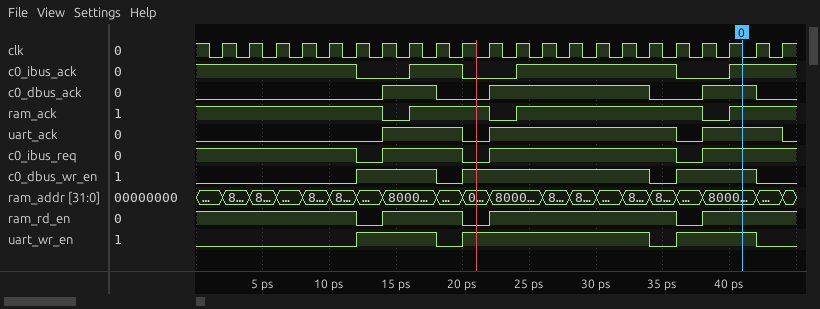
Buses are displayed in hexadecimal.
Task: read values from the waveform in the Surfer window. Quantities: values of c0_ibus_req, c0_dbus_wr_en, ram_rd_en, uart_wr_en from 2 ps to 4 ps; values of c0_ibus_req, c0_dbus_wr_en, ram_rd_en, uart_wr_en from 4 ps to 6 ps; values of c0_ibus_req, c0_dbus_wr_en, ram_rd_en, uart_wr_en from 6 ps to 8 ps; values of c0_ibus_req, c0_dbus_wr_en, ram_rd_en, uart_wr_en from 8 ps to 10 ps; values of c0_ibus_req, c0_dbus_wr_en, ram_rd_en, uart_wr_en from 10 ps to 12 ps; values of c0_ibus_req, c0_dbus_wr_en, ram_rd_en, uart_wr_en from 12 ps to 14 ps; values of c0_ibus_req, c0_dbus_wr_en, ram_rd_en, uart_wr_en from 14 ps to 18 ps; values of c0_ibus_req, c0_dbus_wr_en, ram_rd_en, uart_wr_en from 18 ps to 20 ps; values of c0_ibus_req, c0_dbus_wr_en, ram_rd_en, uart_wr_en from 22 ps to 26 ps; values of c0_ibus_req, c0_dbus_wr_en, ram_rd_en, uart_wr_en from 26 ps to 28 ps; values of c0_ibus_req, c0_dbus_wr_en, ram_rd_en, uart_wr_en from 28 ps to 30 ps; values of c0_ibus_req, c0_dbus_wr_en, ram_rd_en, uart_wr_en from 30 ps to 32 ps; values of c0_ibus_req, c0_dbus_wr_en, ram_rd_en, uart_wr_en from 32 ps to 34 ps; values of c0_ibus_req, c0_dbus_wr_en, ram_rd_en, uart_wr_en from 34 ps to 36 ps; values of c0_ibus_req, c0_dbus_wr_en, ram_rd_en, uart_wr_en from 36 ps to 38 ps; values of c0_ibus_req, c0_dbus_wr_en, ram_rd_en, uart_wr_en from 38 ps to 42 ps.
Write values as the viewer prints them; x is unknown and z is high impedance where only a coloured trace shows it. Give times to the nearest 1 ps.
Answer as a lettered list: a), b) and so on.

a) c0_ibus_req=1, c0_dbus_wr_en=0, ram_rd_en=1, uart_wr_en=0
b) c0_ibus_req=1, c0_dbus_wr_en=0, ram_rd_en=1, uart_wr_en=0
c) c0_ibus_req=1, c0_dbus_wr_en=0, ram_rd_en=1, uart_wr_en=0
d) c0_ibus_req=1, c0_dbus_wr_en=0, ram_rd_en=1, uart_wr_en=0
e) c0_ibus_req=1, c0_dbus_wr_en=0, ram_rd_en=1, uart_wr_en=0
f) c0_ibus_req=0, c0_dbus_wr_en=1, ram_rd_en=0, uart_wr_en=1
g) c0_ibus_req=1, c0_dbus_wr_en=1, ram_rd_en=1, uart_wr_en=1
h) c0_ibus_req=1, c0_dbus_wr_en=0, ram_rd_en=1, uart_wr_en=0
i) c0_ibus_req=1, c0_dbus_wr_en=1, ram_rd_en=1, uart_wr_en=1
j) c0_ibus_req=1, c0_dbus_wr_en=1, ram_rd_en=1, uart_wr_en=1
k) c0_ibus_req=1, c0_dbus_wr_en=1, ram_rd_en=1, uart_wr_en=1
l) c0_ibus_req=1, c0_dbus_wr_en=1, ram_rd_en=1, uart_wr_en=1
m) c0_ibus_req=1, c0_dbus_wr_en=1, ram_rd_en=1, uart_wr_en=1
n) c0_ibus_req=1, c0_dbus_wr_en=0, ram_rd_en=1, uart_wr_en=0
o) c0_ibus_req=0, c0_dbus_wr_en=1, ram_rd_en=0, uart_wr_en=1
p) c0_ibus_req=1, c0_dbus_wr_en=1, ram_rd_en=1, uart_wr_en=1
